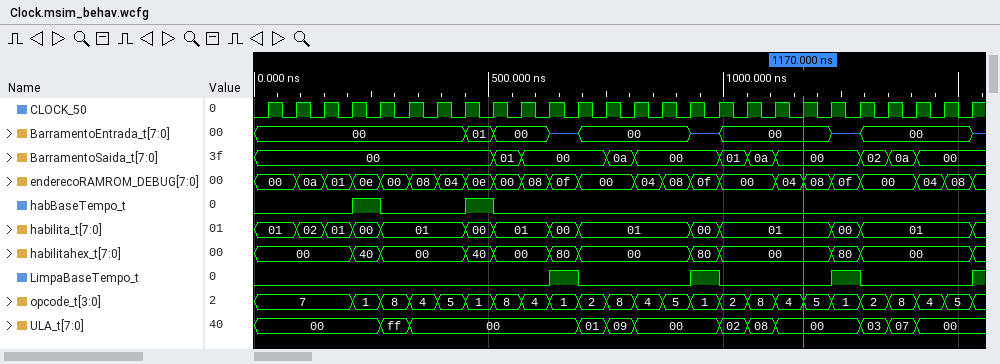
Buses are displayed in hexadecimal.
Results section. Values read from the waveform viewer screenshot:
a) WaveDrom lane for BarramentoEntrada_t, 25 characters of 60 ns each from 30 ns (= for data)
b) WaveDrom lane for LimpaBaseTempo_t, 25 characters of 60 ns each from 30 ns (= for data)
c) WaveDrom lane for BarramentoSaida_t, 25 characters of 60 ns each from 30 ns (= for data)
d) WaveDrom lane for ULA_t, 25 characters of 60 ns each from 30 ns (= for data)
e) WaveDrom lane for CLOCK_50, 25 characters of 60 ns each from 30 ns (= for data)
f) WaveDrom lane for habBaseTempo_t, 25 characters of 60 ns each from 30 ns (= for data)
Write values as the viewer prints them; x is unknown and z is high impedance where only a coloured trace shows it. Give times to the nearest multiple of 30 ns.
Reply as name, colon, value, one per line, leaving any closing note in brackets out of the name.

WaveDrom lane for BarramentoEntrada_t, 25 characters of 60 ns each from 30 ns: {name: 'BarramentoEntrada_t', wave: '=......==.z=...z=...z=...', data: '00 01 00 00 00 00'}
WaveDrom lane for LimpaBaseTempo_t, 25 characters of 60 ns each from 30 ns: {name: 'LimpaBaseTempo_t', wave: '0.........10...10...10...'}
WaveDrom lane for BarramentoSaida_t, 25 characters of 60 ns each from 30 ns: {name: 'BarramentoSaida_t', wave: '=.......==..==..===..===.', data: '00 01 00 0a 00 01 0a 00 02 0a 00'}
WaveDrom lane for ULA_t, 25 characters of 60 ns each from 30 ns: {name: 'ULA_t', wave: '=...==.....===..===..===.', data: '00 ff 00 01 09 00 02 08 00 03 07 00'}
WaveDrom lane for CLOCK_50, 25 characters of 60 ns each from 30 ns: {name: 'CLOCK_50', wave: 'p........................'}
WaveDrom lane for habBaseTempo_t, 25 characters of 60 ns each from 30 ns: {name: 'habBaseTempo_t', wave: '0..10..10................'}
